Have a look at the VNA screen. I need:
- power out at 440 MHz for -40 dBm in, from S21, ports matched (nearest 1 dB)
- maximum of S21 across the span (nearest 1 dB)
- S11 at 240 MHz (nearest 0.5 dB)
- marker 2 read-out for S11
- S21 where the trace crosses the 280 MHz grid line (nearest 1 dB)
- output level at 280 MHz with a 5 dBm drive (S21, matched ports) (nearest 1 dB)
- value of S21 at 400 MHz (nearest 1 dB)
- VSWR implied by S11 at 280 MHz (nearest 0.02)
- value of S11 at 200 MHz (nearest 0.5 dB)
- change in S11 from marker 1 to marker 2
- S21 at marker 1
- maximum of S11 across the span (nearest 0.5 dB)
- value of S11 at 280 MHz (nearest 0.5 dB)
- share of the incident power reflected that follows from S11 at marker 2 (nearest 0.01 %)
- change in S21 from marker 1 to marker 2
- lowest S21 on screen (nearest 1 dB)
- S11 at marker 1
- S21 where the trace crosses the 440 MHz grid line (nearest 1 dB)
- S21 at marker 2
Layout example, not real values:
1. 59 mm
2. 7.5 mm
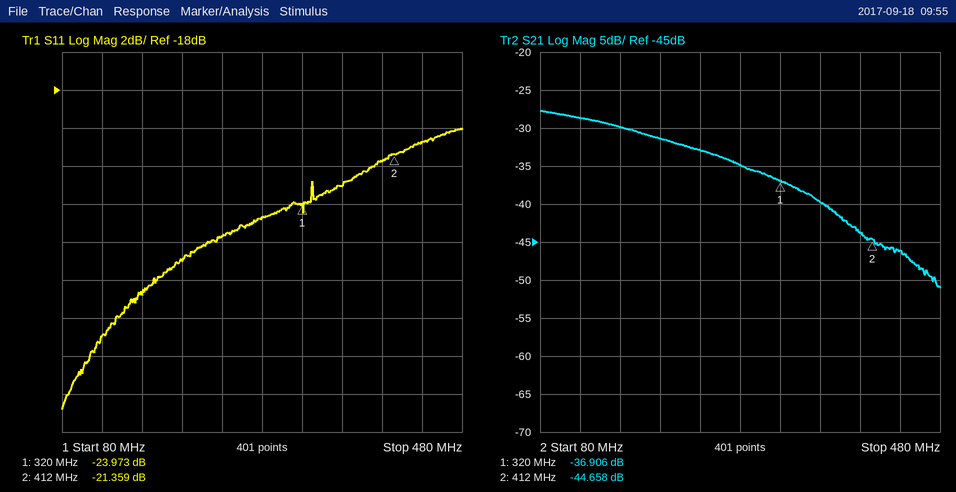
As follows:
1. -86 dBm
2. -28 dB
3. -25.5 dB
4. -21.359 dB
5. -35 dB
6. -30 dBm
7. -44 dB
8. 1.12
9. -27.0 dB
10. 2.614 dB
11. -36.906 dB
12. -20.0 dB
13. -24.5 dB
14. 0.73 %
15. -7.752 dB
16. -51 dB
17. -23.973 dB
18. -46 dB
19. -44.658 dB
